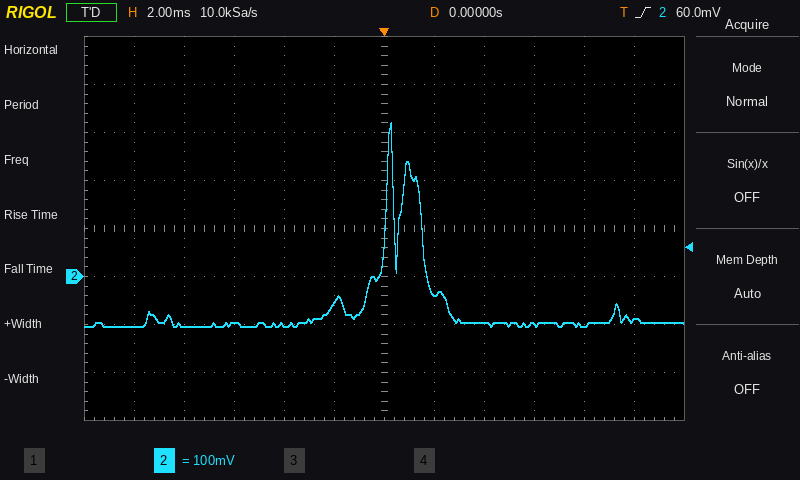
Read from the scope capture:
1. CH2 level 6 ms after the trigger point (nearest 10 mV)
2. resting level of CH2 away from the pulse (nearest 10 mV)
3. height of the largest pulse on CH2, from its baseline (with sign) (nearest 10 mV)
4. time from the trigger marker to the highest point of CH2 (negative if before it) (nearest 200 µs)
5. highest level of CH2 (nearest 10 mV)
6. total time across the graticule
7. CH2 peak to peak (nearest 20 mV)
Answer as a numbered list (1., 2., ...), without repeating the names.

1. -100 mV
2. -100 mV
3. +420 mV
4. +200 µs
5. 320 mV
6. 24 ms
7. 420 mV
